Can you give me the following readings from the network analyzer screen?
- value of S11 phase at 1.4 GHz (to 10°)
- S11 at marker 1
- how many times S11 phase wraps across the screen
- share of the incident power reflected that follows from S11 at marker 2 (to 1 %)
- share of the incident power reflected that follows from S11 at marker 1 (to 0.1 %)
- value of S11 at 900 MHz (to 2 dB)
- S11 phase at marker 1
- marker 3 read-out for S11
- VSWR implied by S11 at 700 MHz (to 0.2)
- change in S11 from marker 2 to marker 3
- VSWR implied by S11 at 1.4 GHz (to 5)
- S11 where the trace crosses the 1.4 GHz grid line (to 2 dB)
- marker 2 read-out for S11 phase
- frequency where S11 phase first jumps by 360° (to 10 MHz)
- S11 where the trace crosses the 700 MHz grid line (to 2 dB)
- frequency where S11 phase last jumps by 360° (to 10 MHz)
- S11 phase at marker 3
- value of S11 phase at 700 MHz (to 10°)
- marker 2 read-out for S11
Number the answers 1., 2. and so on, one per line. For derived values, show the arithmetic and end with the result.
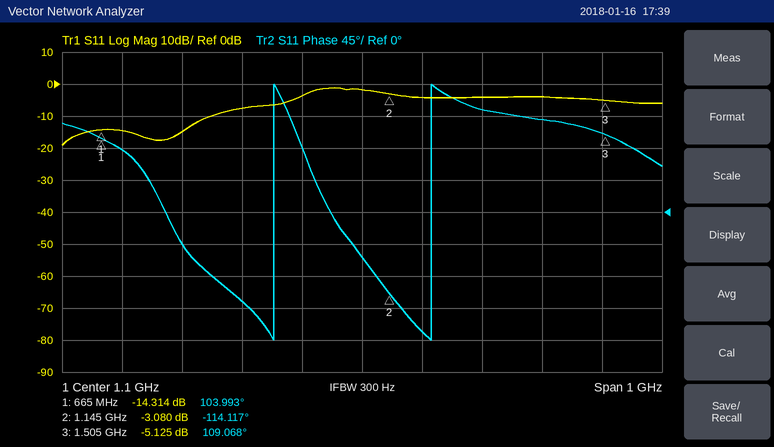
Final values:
1. 130°
2. -14.314 dB
3. 2
4. 10^(-3.08/10) ≈ 49 %
5. 10^(-14.314/10) ≈ 3.7 %
6. -8 dB
7. 103.993°
8. -5.125 dB
9. |Γ| = 10^(-14/20) = 0.1995; VSWR = (1 + 0.1995)/(1 − 0.1995) ≈ 1.50, so 1.4 to the nearest 0.2
10. -5.125 − (-3.08) = -2.045 dB
11. |Γ| = 10^(-4/20) = 0.6310; VSWR = (1 + 0.6310)/(1 − 0.6310) ≈ 4.42, so 5 to the nearest 5
12. -4 dB
13. -114.117°
14. 950 MHz
15. -14 dB
16. 1.22 GHz
17. 109.068°
18. 90°
19. -3.080 dB
